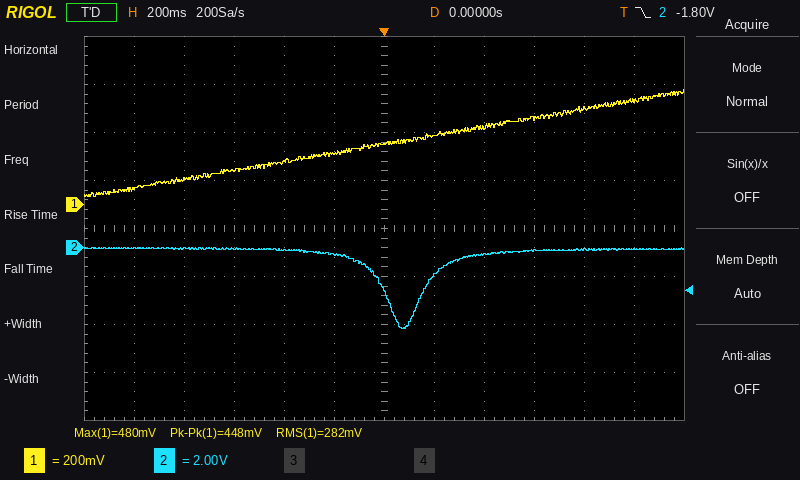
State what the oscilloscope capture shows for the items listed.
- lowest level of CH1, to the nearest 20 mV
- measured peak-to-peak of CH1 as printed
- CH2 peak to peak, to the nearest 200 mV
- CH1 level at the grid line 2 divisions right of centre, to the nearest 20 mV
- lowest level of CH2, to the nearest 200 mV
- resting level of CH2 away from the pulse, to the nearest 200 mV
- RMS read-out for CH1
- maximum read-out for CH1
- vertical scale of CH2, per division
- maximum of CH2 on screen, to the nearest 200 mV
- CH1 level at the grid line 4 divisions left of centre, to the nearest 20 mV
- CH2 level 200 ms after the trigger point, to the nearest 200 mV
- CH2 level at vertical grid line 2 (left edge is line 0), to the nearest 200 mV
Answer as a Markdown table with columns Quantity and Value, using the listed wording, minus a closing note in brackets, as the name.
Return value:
| Quantity | Value |
|---|---|
| lowest level of CH1, to the nearest 20 mV | 40 mV |
| measured peak-to-peak of CH1 as printed | 448 mV |
| CH2 peak to peak, to the nearest 200 mV | 3.4 V |
| CH1 level at the grid line 2 divisions right of centre, to the nearest 20 mV | 320 mV |
| lowest level of CH2, to the nearest 200 mV | -3.4 V |
| resting level of CH2 away from the pulse, to the nearest 200 mV | 0.0 V |
| RMS read-out for CH1 | 282 mV |
| maximum read-out for CH1 | 480 mV |
| vertical scale of CH2, per division | 2 V |
| maximum of CH2 on screen, to the nearest 200 mV | 0.0 V |
| CH1 level at the grid line 4 divisions left of centre, to the nearest 20 mV | 100 mV |
| CH2 level 200 ms after the trigger point, to the nearest 200 mV | -1.2 V |
| CH2 level at vertical grid line 2 (left edge is line 0), to the nearest 200 mV | 0.0 V |
